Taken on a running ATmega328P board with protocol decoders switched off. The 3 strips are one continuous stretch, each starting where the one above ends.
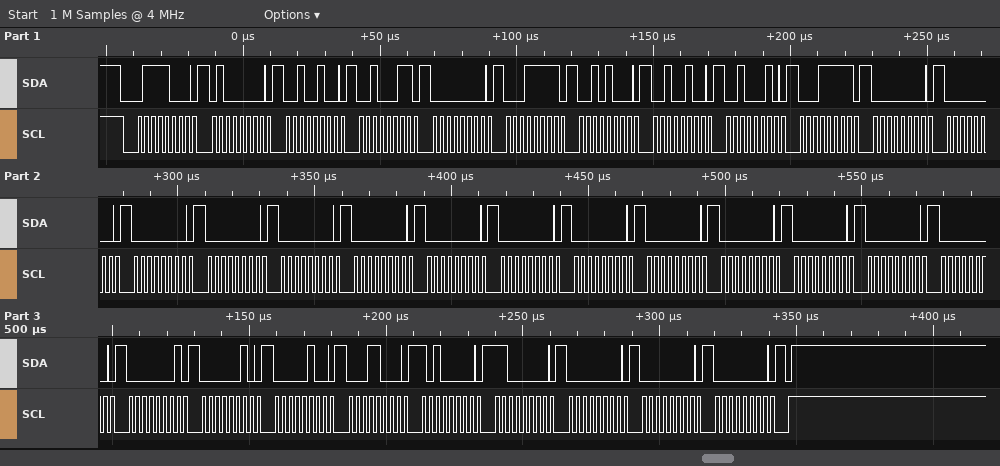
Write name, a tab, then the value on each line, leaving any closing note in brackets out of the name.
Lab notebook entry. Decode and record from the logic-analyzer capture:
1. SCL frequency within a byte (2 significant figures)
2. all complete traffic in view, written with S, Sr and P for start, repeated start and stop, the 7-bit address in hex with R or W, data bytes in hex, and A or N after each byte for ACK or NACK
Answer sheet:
SCL frequency within a byte	400 kHz
all complete traffic in view, written with S, Sr and P for start, repeated start and stop, the 7-bit address in hex with R or W, data bytes in hex, and A or N after each byte for ACK or NACK	S 3CW A 40 A 24 A 23 A 00 A 1F A 28 A 24 A 22 A 1F A 00 A 00 A 00 A 00 A 00 A 00 A 00 A 00 A 00 A 00 A 00 A 00 A 00 A 00 A 01 A 02 A 04 A 18 A A0 A C0 A 00 A 00 A 00 A P
